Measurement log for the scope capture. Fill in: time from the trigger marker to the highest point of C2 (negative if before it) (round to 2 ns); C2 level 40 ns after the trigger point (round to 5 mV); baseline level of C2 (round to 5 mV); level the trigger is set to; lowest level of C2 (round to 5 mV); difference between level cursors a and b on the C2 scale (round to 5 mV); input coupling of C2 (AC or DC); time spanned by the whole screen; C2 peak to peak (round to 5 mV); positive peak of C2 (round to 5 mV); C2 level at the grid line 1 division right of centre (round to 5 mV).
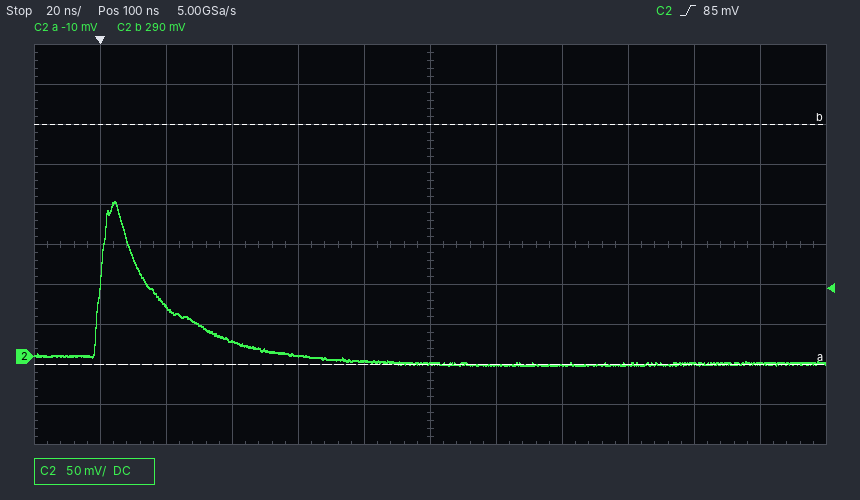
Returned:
+4 ns
20 mV
-10 mV
85 mV
-10 mV
300 mV
DC
240 ns
205 mV
195 mV
-10 mV
